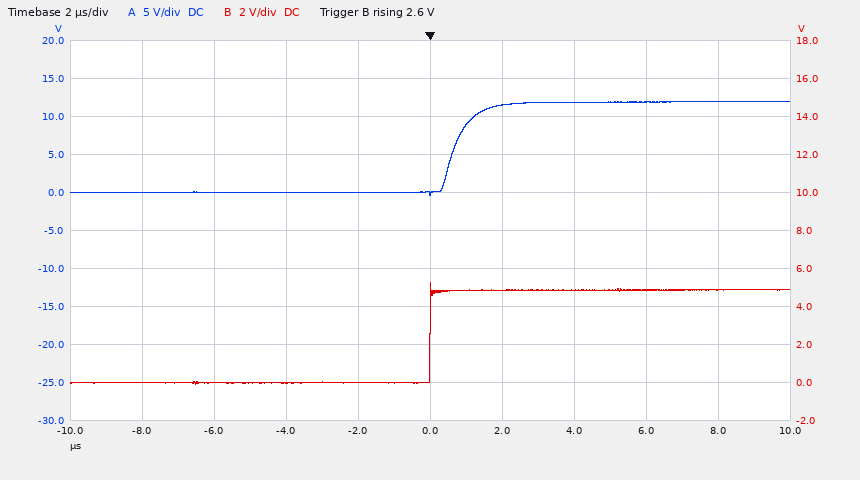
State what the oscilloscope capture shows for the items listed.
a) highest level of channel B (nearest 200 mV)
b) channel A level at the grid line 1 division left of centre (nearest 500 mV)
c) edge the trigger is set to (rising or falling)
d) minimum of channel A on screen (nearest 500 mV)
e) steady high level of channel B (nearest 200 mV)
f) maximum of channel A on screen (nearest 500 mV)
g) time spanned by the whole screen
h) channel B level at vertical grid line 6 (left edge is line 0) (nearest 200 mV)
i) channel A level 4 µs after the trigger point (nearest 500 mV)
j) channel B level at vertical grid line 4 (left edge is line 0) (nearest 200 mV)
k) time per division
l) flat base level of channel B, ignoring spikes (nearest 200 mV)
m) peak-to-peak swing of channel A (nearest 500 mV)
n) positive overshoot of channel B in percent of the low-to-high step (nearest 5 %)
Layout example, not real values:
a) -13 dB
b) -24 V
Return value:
a) 5.2 V
b) 0.0 V
c) rising
d) -500 mV
e) 4.8 V
f) 12.0 V
g) 20 µs
h) 4.8 V
i) 12.0 V
j) 0.0 V
k) 2 µs
l) 0.0 V
m) 12.5 V
n) 10 %
